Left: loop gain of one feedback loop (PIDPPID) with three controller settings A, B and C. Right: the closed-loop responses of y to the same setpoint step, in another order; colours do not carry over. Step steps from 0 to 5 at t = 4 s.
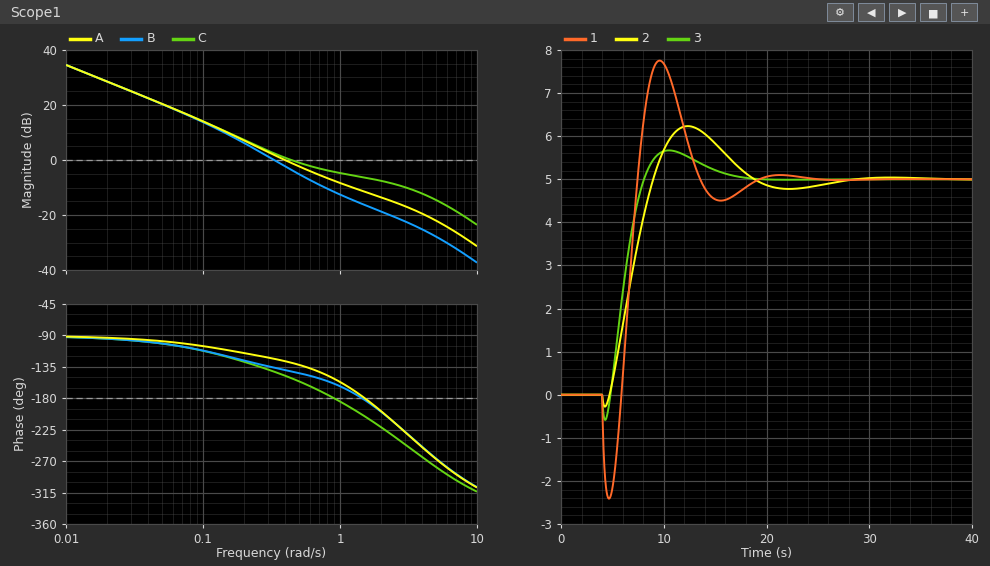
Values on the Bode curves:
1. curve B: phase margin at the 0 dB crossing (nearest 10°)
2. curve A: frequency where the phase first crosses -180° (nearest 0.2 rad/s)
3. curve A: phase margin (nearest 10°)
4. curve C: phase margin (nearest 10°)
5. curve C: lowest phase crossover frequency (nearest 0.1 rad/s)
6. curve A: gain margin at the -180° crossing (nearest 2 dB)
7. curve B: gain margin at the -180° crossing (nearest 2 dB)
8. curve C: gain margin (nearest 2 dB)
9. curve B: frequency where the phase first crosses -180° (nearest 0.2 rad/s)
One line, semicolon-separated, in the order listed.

40°; 1.6 rad/s; 50°; 30°; 0.9 rad/s; 12 dB; 16 dB; 4 dB; 1.4 rad/s
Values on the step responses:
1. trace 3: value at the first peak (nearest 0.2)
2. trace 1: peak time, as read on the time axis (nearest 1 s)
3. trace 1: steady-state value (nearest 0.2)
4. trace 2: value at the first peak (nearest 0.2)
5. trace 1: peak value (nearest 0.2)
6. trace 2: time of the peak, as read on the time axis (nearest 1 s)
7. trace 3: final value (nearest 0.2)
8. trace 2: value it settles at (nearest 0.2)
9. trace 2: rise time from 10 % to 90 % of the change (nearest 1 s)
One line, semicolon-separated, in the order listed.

5.6; 10 s; 5.0; 6.2; 7.8; 12 s; 5.0; 5.0; 3 s
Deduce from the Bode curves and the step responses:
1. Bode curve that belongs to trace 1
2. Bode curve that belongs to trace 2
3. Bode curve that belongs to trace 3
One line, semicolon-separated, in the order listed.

C; B; A
